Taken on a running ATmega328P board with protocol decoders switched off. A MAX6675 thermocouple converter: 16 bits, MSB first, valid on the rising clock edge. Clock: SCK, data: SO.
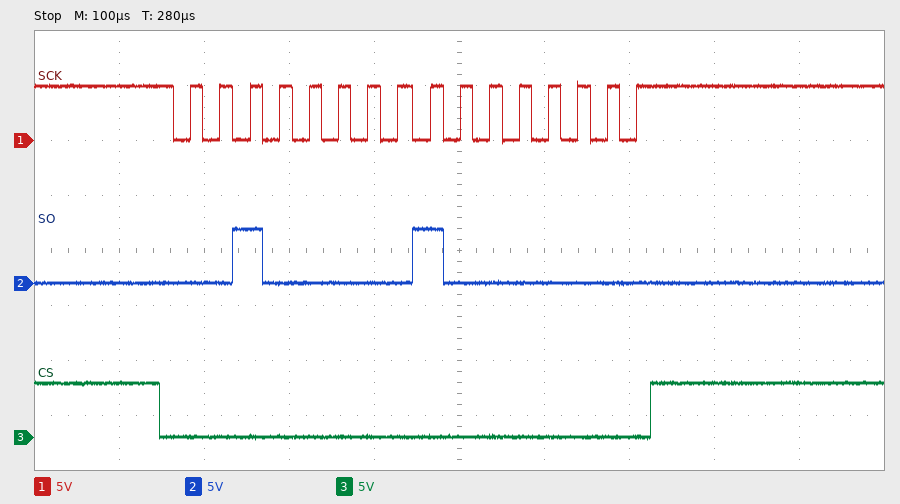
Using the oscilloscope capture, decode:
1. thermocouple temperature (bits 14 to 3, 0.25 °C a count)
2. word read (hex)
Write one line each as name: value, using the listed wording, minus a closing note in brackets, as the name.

thermocouple temperature: 260.00 °C
word read: 0x2080
